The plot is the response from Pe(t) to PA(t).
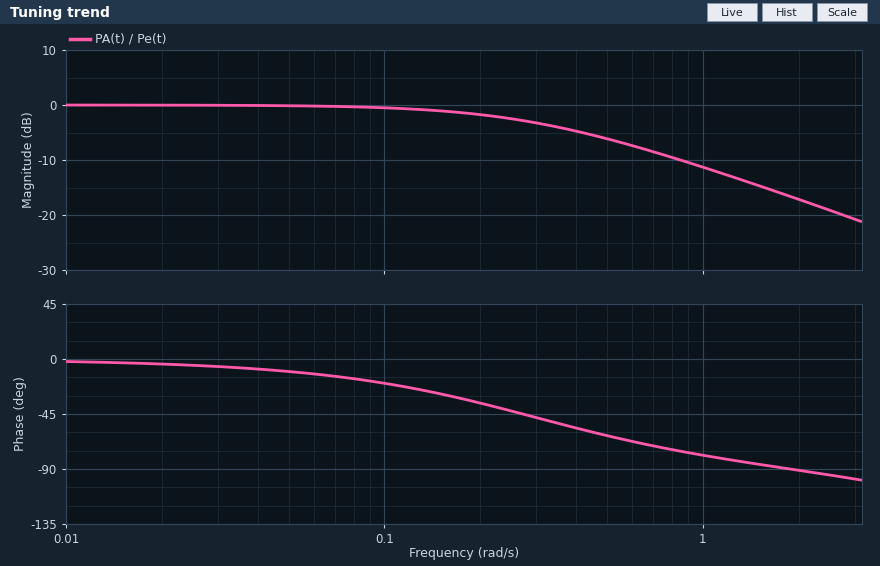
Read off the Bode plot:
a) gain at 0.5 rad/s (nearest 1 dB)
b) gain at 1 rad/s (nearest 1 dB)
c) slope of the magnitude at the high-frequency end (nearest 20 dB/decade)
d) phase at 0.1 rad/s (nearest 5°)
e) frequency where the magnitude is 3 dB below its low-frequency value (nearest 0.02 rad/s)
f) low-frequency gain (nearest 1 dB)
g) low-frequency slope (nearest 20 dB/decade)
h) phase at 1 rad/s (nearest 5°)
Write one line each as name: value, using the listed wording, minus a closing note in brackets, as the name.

gain at 0.5 rad/s: -6 dB
gain at 1 rad/s: -11 dB
slope of the magnitude at the high-frequency end: -20 dB/decade
phase at 0.1 rad/s: -20°
frequency where the magnitude is 3 dB below its low-frequency value: 0.28 rad/s
low-frequency gain: 0 dB
low-frequency slope: 0 dB/decade
phase at 1 rad/s: -80°
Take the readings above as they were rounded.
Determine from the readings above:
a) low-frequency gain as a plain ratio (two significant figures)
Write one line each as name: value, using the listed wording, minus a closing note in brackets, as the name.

low-frequency gain as a plain ratio: 1.0
